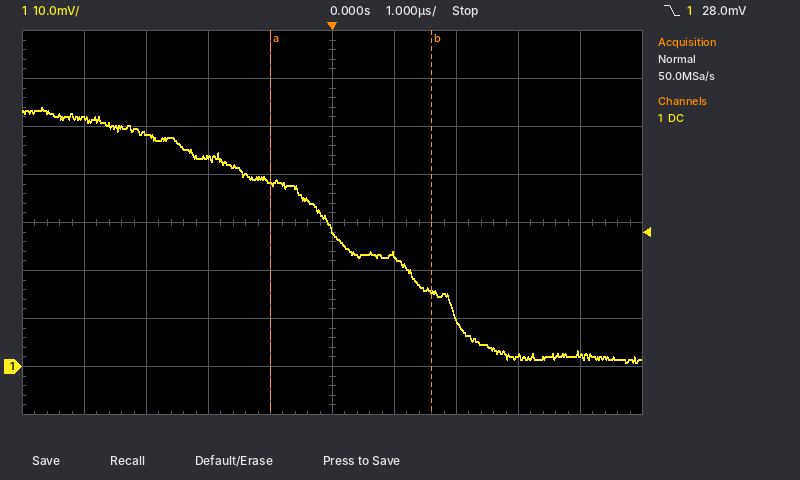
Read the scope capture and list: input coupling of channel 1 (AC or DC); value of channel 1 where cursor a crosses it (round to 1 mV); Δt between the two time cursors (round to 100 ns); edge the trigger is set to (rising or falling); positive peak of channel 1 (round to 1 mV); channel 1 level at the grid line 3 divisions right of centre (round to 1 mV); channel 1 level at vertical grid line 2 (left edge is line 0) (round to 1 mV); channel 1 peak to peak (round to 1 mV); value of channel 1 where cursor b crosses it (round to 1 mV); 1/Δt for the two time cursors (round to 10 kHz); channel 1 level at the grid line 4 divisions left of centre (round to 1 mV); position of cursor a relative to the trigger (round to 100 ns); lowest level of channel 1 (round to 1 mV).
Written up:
DC
38 mV
2.6 µs
falling
54 mV
2 mV
49 mV
53 mV
16 mV
380 kHz
52 mV
-1.0 µs
1 mV
